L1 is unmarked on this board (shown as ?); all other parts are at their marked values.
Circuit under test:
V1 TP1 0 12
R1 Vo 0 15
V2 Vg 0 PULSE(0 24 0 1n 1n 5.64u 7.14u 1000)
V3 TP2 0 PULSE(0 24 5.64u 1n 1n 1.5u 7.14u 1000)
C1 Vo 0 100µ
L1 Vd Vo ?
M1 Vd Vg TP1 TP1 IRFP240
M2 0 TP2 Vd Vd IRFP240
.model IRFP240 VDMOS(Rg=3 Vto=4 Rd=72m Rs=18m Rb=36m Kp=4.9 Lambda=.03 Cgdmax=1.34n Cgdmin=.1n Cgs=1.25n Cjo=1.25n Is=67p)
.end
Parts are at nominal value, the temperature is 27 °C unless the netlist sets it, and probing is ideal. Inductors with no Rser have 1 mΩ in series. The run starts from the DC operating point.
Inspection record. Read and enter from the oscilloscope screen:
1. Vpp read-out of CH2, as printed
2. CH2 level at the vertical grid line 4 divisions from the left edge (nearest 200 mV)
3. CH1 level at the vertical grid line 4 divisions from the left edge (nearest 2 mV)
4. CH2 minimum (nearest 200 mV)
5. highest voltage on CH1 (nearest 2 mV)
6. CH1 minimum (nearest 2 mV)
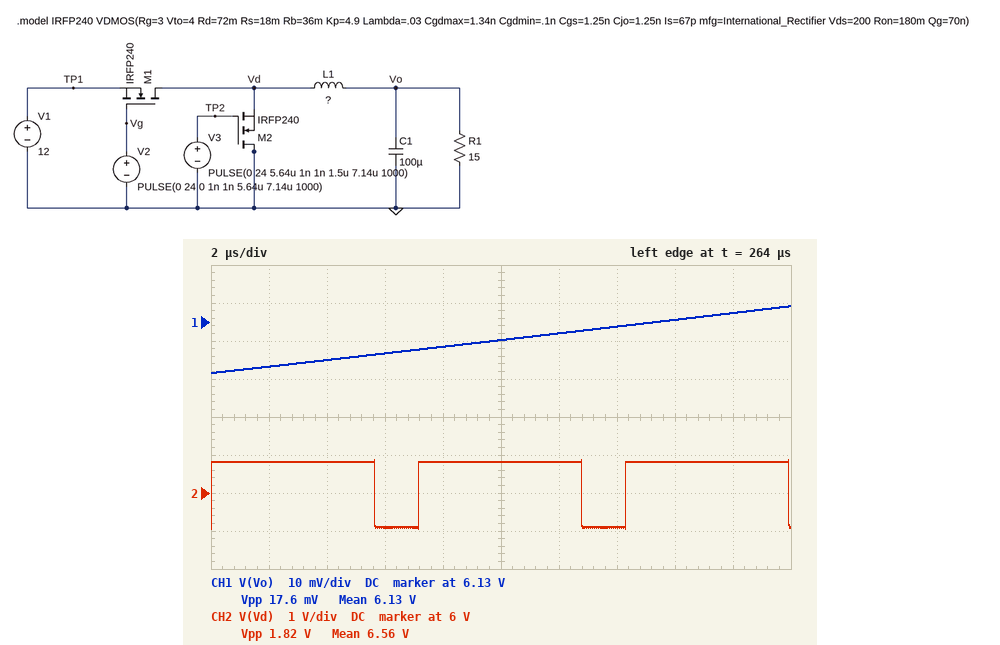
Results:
1.82 V
6.8 V
6.124 V
5.0 V
6.134 V
6.116 V
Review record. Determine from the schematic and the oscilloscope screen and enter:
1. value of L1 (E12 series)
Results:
1.2 mH
